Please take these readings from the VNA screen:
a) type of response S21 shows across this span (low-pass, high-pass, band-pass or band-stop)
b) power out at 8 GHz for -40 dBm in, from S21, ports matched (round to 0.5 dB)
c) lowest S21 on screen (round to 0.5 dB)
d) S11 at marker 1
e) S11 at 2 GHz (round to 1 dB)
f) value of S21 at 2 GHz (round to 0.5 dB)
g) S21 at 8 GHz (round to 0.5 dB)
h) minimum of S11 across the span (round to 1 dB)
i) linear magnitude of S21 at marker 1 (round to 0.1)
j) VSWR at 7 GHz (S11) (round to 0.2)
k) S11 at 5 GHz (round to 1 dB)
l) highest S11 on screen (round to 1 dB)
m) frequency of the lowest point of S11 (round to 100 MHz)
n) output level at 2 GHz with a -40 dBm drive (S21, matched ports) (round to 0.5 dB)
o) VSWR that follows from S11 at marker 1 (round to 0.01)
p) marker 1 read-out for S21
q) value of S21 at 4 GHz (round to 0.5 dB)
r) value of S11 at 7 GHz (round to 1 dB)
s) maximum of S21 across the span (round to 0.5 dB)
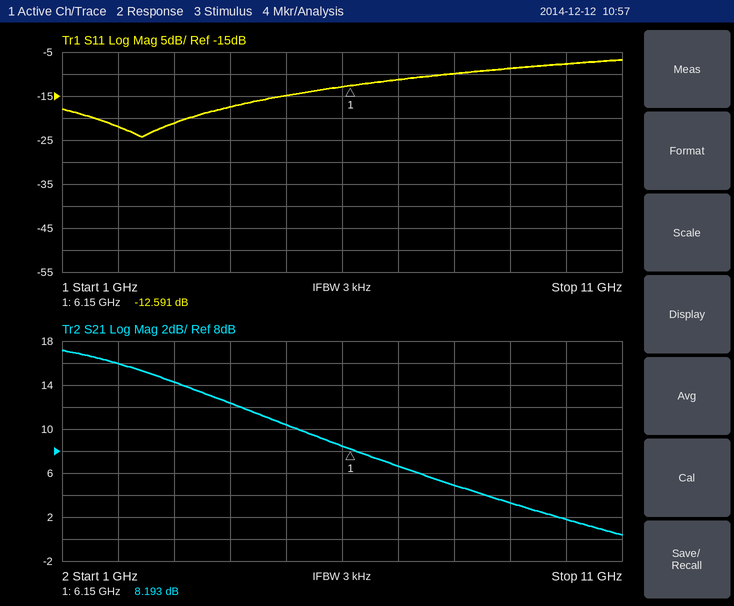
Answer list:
low-pass
-35.0 dBm
0.5 dB
-12.591 dB
-22 dB
16.0 dB
5.0 dB
-24 dB
2.6
1.8
-15 dB
-7 dB
2.4 GHz
-24.0 dBm
1.61
8.193 dB
12.5 dB
-11 dB
17.0 dB
